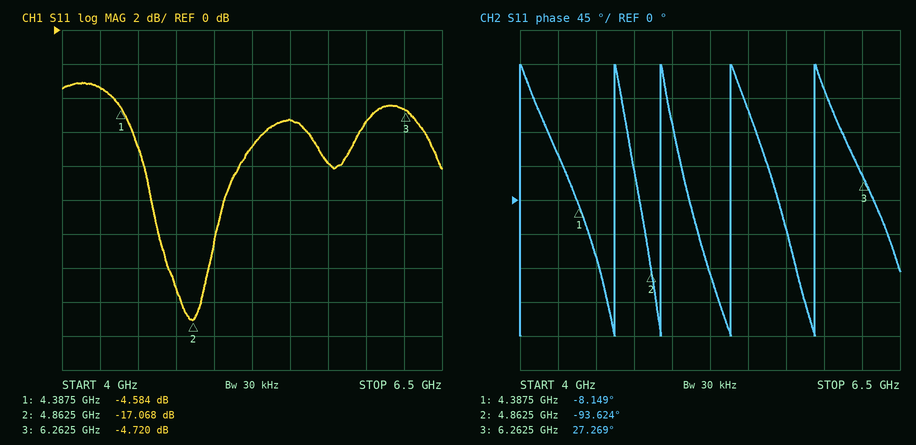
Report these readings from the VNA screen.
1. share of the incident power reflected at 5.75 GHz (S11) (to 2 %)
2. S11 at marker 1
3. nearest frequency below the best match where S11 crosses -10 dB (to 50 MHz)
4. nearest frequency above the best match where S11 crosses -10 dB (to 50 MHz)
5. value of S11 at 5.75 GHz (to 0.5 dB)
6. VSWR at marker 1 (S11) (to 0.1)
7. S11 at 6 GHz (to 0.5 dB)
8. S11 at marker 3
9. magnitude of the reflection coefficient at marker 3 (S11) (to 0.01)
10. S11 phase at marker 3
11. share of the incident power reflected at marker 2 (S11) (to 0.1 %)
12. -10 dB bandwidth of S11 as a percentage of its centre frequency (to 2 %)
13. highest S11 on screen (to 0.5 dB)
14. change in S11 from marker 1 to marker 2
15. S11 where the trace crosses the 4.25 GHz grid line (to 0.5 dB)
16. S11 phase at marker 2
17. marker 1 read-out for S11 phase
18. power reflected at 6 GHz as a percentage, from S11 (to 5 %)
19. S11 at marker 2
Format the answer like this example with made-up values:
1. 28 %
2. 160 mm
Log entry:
1. 16 %
2. -4.584 dB
3. 4.60 GHz
4. 5.05 GHz
5. -8.0 dB
6. 3.9
7. -5.5 dB
8. -4.720 dB
9. 0.58
10. 27.269°
11. 2.0 %
12. 10 %
13. -3.0 dB
14. -12.484 dB
15. -3.5 dB
16. -93.624°
17. -8.149°
18. 30 %
19. -17.068 dB
